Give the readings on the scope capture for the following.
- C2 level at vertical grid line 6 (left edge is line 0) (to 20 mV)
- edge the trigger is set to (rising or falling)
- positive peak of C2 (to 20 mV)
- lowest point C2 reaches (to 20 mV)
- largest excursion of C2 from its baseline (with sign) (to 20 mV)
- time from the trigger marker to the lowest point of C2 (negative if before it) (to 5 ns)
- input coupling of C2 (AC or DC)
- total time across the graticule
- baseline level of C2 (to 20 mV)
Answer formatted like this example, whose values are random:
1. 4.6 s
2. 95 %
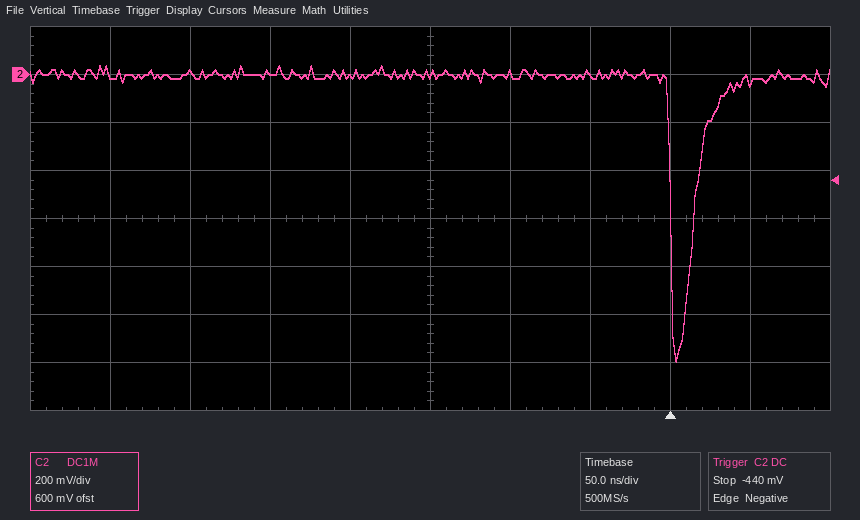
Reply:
1. 0 mV
2. falling
3. 40 mV
4. -1.20 V
5. -1.20 V
6. +5 ns
7. DC
8. 500 ns
9. 0 mV
